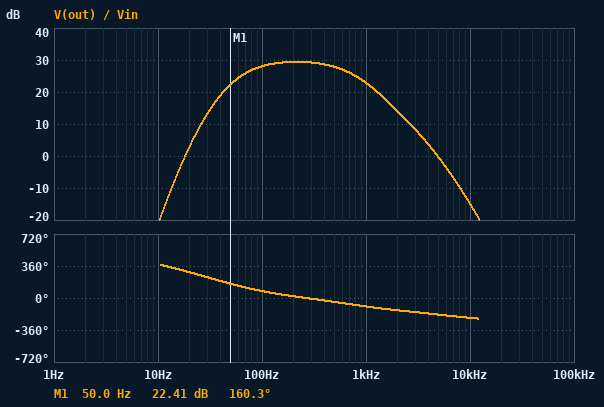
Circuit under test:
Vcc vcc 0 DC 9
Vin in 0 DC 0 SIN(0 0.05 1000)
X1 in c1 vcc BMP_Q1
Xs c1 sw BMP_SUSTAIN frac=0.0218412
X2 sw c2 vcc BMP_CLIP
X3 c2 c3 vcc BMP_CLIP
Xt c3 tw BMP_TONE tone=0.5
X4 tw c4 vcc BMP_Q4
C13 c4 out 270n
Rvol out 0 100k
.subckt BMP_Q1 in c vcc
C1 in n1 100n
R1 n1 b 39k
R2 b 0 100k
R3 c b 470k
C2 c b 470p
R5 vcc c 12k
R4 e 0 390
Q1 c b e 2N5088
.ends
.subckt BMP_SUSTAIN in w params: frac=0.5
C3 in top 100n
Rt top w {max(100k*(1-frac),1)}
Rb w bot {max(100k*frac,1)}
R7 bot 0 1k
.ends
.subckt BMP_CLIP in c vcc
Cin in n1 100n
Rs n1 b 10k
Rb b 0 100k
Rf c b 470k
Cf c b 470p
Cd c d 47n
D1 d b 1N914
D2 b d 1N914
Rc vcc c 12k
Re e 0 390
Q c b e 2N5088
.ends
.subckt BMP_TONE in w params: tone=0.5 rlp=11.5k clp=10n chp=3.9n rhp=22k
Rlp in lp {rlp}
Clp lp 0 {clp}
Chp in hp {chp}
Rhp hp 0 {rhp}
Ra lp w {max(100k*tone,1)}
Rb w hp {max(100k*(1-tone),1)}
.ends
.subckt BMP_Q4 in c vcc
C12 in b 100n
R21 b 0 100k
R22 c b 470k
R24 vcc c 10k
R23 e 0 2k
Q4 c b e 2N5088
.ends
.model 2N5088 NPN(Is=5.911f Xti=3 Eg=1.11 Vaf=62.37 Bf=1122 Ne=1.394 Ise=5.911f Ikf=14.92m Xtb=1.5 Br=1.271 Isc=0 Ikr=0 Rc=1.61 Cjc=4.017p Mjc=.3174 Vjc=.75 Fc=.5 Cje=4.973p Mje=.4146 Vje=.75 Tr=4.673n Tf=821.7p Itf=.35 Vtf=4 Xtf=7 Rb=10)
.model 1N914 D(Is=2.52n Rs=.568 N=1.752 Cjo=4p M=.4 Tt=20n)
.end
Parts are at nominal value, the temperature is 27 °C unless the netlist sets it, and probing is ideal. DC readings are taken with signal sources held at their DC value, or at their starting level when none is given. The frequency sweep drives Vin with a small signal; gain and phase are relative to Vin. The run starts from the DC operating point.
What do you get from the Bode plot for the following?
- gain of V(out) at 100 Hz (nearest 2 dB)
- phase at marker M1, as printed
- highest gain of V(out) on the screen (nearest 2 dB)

28 dB
160.3 deg
30 dB
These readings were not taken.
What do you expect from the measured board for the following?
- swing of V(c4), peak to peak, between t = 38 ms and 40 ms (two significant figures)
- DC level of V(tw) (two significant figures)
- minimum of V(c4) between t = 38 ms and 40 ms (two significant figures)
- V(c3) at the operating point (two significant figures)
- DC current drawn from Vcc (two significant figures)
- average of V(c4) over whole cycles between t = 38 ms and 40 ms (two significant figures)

700 mV
2.5 V
6.2 V
4.6 V
1.3 mA
6.5 V
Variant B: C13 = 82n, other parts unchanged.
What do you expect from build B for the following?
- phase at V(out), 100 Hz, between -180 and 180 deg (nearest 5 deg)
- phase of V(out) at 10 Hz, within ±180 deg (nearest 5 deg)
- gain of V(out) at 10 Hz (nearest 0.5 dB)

85 deg
50 deg
-26.5 dB
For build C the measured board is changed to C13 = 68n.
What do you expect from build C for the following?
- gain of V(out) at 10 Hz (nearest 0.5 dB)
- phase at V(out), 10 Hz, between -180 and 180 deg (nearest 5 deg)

-28.0 dB
55 deg
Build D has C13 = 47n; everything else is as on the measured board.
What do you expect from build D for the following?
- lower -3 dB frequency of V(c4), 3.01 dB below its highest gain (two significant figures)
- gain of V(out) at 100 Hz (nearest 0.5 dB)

73 Hz
27.5 dB
